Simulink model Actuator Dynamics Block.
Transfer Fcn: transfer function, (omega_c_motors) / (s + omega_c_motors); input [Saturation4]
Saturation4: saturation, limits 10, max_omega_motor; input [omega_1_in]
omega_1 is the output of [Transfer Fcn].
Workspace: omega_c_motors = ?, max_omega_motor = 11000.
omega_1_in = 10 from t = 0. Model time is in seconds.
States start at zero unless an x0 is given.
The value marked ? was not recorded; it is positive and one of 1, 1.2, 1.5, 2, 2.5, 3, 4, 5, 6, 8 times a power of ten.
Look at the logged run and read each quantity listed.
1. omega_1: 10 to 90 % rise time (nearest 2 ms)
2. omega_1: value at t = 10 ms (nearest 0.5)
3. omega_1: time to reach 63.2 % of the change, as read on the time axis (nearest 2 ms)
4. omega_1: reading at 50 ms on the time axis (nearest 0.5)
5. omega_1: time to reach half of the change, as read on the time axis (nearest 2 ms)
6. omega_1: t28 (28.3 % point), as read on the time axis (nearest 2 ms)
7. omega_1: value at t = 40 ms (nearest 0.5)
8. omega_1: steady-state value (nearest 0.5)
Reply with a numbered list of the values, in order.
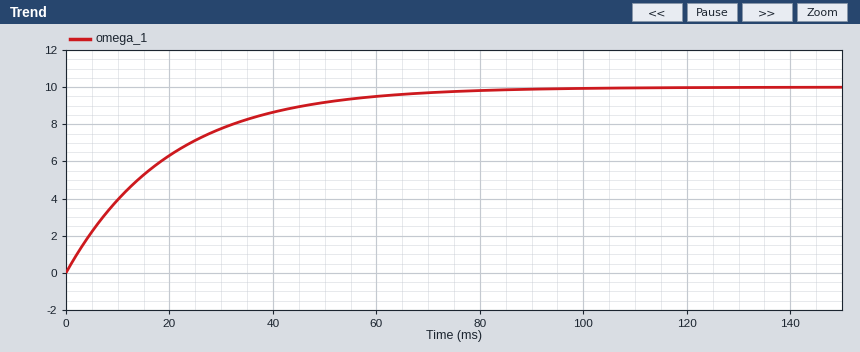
1. 44 ms
2. 4.0
3. 20 ms
4. 9.0
5. 14 ms
6. 6 ms
7. 8.5
8. 10.0
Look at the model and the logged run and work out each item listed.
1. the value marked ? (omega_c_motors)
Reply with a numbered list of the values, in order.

1. 50
